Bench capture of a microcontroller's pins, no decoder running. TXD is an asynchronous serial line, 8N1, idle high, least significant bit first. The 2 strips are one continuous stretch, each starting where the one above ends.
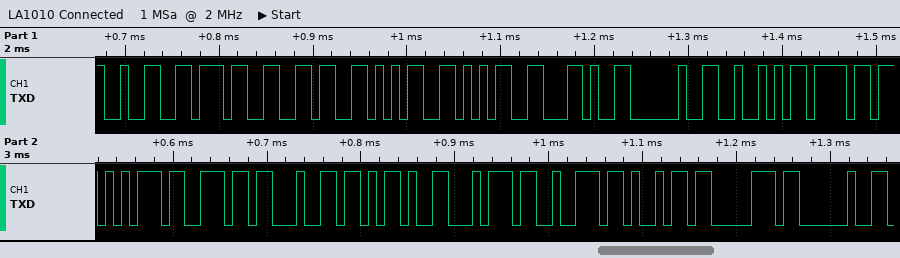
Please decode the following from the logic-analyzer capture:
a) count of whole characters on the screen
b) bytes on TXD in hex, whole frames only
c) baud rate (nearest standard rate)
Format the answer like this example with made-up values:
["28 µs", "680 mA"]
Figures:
["18", "0x32 0x37 0x36 0x35 0x35 0x2C 0x20 0x52 0x6F 0x75 0x6E 0x64 0x2D 0x74 0x72 0x69 0x70 0x20", "115200 baud"]
